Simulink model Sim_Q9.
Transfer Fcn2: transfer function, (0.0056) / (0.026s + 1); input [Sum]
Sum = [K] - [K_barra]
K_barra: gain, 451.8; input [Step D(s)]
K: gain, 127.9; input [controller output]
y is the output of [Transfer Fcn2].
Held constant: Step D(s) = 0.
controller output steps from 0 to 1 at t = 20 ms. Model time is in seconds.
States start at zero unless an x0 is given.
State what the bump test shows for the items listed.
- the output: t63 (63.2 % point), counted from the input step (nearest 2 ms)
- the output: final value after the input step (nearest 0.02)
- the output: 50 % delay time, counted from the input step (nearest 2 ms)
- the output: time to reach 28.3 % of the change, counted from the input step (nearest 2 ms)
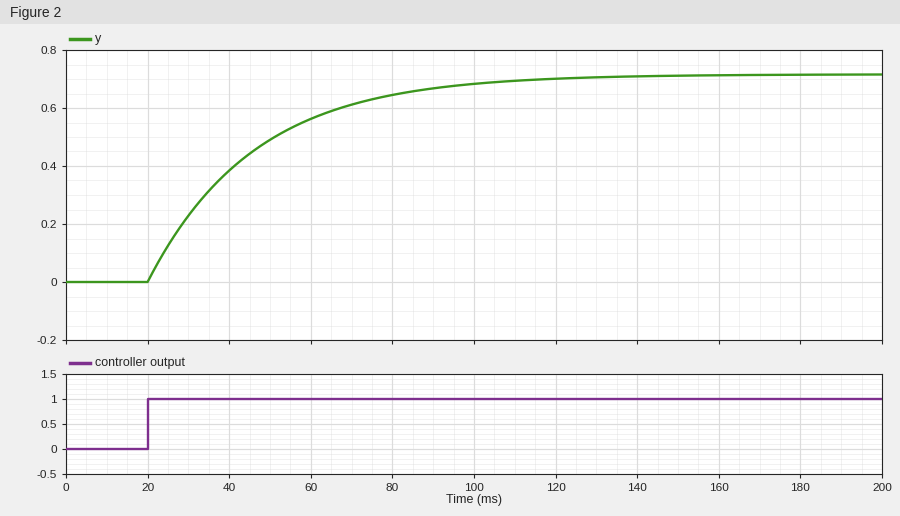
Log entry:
26 ms
0.72
18 ms
8 ms
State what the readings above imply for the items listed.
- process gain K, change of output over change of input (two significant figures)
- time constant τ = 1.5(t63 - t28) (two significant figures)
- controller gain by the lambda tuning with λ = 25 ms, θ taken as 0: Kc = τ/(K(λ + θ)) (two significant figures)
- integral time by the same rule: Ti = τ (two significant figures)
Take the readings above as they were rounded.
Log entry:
0.72
27 ms
1.5
27 ms
